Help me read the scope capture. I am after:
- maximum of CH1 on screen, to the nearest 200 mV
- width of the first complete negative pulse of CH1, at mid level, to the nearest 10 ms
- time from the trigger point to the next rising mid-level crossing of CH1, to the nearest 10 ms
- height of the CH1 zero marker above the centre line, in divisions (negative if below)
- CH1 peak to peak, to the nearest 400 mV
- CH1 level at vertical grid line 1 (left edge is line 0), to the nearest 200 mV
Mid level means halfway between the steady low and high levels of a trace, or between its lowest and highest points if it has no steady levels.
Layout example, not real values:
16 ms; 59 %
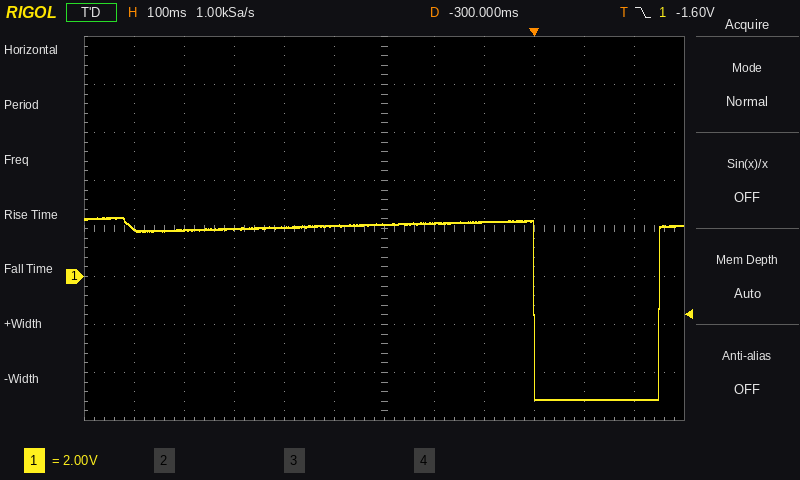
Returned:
2.4 V; 250 ms; 250 ms; -1.0 div; 7.6 V; 2.0 V
